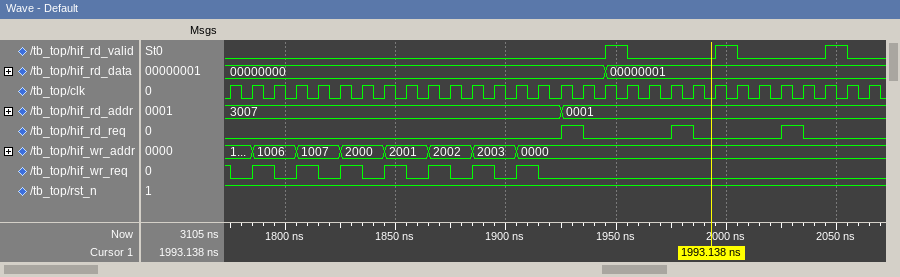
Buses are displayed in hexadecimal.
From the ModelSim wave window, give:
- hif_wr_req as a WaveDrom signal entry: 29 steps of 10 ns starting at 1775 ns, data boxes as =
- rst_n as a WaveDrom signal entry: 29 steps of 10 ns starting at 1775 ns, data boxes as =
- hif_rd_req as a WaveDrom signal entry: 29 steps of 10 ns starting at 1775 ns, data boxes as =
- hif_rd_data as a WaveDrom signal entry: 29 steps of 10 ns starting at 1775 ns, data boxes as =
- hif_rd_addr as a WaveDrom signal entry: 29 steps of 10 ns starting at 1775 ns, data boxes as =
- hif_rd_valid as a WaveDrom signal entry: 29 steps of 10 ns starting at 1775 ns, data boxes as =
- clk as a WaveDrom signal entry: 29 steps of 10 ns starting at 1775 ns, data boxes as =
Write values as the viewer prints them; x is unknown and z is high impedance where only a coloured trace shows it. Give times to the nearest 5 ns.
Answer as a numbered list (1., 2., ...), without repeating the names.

1. {name: 'hif_wr_req', wave: '010101010101010..............'}
2. {name: 'rst_n', wave: '1............................'}
3. {name: 'hif_rd_req', wave: '0..............10...10...10..'}
4. {name: 'hif_rd_data', wave: '=................=...........', data: '00000000 00000001'}
5. {name: 'hif_rd_addr', wave: '=..............=.............', data: '3007 0001'}
6. {name: 'hif_rd_valid', wave: '0................10...10...10'}
7. {name: 'clk', wave: 'p............................'}
